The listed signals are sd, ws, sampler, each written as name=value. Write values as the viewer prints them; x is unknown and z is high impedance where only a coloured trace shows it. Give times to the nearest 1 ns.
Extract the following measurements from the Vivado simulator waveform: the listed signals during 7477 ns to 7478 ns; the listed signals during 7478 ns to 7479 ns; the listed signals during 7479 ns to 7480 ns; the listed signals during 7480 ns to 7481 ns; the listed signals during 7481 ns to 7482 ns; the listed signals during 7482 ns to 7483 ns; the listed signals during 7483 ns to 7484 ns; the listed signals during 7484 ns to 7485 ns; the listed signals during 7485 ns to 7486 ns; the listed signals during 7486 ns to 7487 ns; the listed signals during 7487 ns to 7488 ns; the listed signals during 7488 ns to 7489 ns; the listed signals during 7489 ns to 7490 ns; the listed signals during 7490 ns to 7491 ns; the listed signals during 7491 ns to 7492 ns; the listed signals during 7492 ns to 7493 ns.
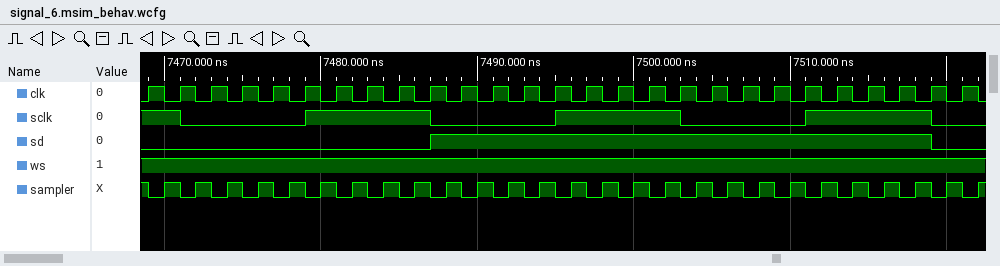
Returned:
sd=0, ws=1, sampler=0
sd=0, ws=1, sampler=1
sd=0, ws=1, sampler=0
sd=0, ws=1, sampler=1
sd=0, ws=1, sampler=0
sd=0, ws=1, sampler=1
sd=0, ws=1, sampler=0
sd=0, ws=1, sampler=1
sd=0, ws=1, sampler=0
sd=0, ws=1, sampler=1
sd=1, ws=1, sampler=0
sd=1, ws=1, sampler=1
sd=1, ws=1, sampler=0
sd=1, ws=1, sampler=1
sd=1, ws=1, sampler=0
sd=1, ws=1, sampler=1
